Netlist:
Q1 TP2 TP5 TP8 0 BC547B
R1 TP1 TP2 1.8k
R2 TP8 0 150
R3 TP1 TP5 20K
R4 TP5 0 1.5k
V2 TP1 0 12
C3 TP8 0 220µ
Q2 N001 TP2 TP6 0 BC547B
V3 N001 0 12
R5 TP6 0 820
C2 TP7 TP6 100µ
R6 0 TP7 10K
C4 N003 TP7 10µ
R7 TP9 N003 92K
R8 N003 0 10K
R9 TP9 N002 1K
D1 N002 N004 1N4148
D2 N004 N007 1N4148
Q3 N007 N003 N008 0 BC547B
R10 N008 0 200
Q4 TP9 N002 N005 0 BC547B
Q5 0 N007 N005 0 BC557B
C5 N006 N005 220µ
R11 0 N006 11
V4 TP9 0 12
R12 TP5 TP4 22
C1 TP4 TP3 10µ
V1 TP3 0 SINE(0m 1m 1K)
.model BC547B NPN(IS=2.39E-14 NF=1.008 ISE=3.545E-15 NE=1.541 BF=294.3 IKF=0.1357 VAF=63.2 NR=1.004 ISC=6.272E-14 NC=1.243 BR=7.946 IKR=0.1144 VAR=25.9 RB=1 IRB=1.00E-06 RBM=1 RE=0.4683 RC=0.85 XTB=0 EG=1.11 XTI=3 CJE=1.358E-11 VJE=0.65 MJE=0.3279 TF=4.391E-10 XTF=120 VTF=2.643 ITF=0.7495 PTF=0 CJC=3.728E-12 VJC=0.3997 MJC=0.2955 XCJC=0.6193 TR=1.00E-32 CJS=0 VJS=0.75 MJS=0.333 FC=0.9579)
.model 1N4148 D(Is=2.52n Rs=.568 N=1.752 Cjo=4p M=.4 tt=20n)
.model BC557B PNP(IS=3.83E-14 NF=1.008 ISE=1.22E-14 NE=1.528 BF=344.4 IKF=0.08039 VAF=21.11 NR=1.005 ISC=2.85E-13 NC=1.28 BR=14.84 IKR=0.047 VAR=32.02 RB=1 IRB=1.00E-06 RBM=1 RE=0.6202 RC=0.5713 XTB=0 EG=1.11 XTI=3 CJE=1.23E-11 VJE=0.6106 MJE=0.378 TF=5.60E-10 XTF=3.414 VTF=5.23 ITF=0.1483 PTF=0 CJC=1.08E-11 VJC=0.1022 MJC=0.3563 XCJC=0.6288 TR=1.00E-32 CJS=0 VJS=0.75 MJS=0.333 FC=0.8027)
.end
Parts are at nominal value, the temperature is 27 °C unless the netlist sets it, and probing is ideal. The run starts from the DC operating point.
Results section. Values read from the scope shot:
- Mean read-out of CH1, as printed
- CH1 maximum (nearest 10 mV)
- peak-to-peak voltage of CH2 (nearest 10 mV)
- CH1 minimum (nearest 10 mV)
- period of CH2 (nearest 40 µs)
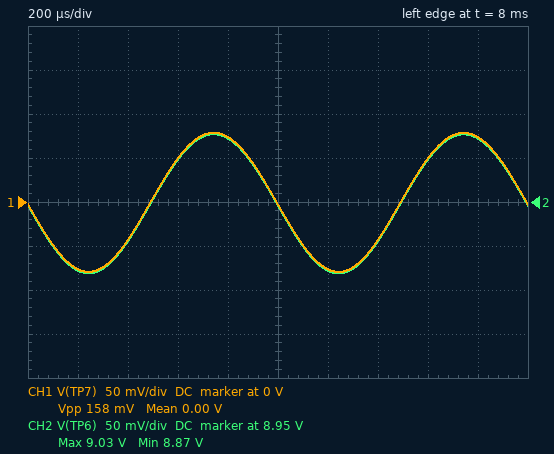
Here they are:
0.00 V
80 mV
160 mV
-80 mV
1.00 ms
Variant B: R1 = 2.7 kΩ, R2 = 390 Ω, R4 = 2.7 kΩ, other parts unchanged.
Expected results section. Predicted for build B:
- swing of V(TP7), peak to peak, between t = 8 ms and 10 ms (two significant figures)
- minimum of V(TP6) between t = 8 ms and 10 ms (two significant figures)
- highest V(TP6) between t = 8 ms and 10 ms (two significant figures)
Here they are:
340 mV
5.8 V
6.2 V
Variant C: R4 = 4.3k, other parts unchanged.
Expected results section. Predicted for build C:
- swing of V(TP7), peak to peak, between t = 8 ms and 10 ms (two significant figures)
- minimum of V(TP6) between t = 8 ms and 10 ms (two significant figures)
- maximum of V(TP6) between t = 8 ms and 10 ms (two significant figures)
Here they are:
6.7 mV
390 mV
400 mV
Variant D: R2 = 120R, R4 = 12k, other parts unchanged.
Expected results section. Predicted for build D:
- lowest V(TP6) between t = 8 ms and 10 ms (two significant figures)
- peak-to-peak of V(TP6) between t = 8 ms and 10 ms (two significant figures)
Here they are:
240 mV
1.7 mV
